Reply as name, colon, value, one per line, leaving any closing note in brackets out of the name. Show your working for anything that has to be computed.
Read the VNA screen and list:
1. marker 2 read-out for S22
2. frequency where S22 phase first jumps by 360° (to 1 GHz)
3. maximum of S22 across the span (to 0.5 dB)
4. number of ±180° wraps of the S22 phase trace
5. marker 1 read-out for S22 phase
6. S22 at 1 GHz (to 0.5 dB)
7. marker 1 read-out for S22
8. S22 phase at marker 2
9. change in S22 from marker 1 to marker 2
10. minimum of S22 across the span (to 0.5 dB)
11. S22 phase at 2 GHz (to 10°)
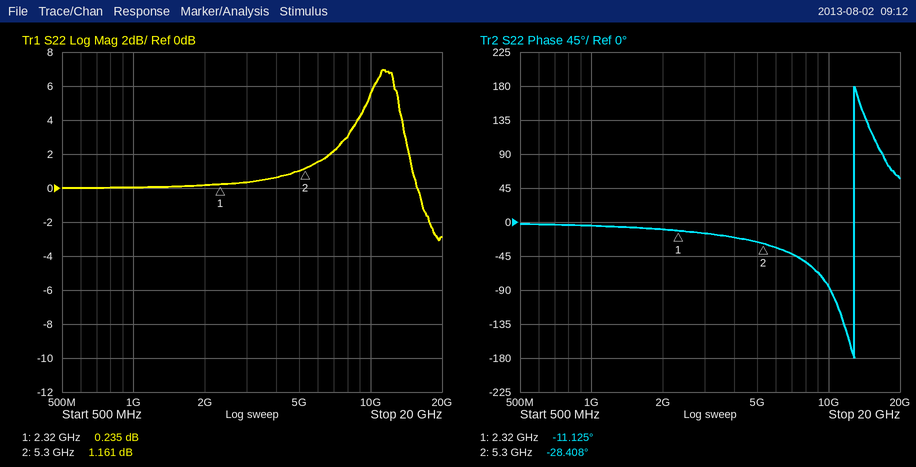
marker 2 read-out for S22: 1.161 dB
frequency where S22 phase first jumps by 360°: 13 GHz
maximum of S22 across the span: 7.0 dB
number of ±180° wraps of the S22 phase trace: 1
marker 1 read-out for S22 phase: -11.125°
S22 at 1 GHz: 0.0 dB
marker 1 read-out for S22: 0.235 dB
S22 phase at marker 2: -28.408°
change in S22 from marker 1 to marker 2: 1.161 − (0.235) = 0.926 dB
minimum of S22 across the span: -3.0 dB
S22 phase at 2 GHz: -10°
